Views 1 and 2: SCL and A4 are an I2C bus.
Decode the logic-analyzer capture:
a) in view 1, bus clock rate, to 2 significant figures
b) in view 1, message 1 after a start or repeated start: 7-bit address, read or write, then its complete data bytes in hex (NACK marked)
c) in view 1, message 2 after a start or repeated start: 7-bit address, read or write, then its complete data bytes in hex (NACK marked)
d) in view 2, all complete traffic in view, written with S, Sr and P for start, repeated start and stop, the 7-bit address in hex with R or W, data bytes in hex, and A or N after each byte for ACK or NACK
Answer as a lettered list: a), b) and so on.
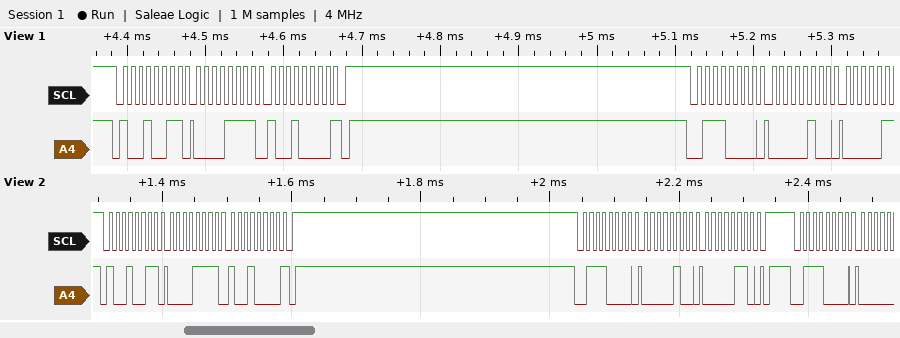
a) 100 kHz
b) 0x49 read: 0F 90 NACK
c) 0x38 write: 04
d) S 49R A 0F A 90 N P S 38W A 04 A 06 A P S 38W A
